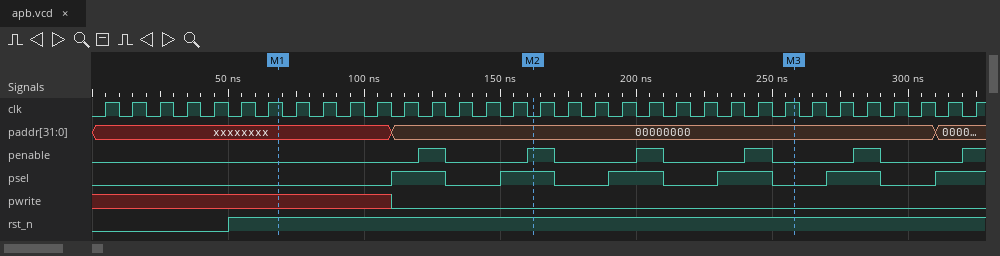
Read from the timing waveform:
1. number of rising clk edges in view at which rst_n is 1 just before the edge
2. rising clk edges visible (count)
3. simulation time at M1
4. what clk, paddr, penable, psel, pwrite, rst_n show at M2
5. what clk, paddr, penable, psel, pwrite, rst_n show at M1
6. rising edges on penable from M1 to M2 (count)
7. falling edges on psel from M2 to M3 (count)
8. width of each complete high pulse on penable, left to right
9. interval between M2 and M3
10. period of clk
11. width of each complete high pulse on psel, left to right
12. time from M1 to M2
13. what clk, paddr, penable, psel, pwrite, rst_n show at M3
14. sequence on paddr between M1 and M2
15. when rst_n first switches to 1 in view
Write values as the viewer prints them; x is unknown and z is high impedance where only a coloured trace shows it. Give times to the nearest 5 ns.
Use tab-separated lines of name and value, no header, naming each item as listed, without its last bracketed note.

number of rising clk edges in view at which rst_n is 1 just before the edge	28
rising clk edges visible	33
simulation time at M1	70 ns
what clk, paddr, penable, psel, pwrite, rst_n show at M2	clk=0, paddr=00000000, penable=1, psel=1, pwrite=0, rst_n=1
what clk, paddr, penable, psel, pwrite, rst_n show at M1	clk=1, paddr=xxxxxxxx, penable=0, psel=0, pwrite=x, rst_n=1
rising edges on penable from M1 to M2	2
falling edges on psel from M2 to M3	3
width of each complete high pulse on penable, left to right	10 ns, 10 ns, 10 ns, 10 ns, 10 ns
interval between M2 and M3	95 ns
period of clk	10 ns
width of each complete high pulse on psel, left to right	20 ns, 20 ns, 20 ns, 20 ns, 20 ns
time from M1 to M2	95 ns
what clk, paddr, penable, psel, pwrite, rst_n show at M3	clk=1, paddr=00000000, penable=0, psel=0, pwrite=0, rst_n=1
sequence on paddr between M1 and M2	xxxxxxxx, 00000000
when rst_n first switches to 1 in view	50 ns
